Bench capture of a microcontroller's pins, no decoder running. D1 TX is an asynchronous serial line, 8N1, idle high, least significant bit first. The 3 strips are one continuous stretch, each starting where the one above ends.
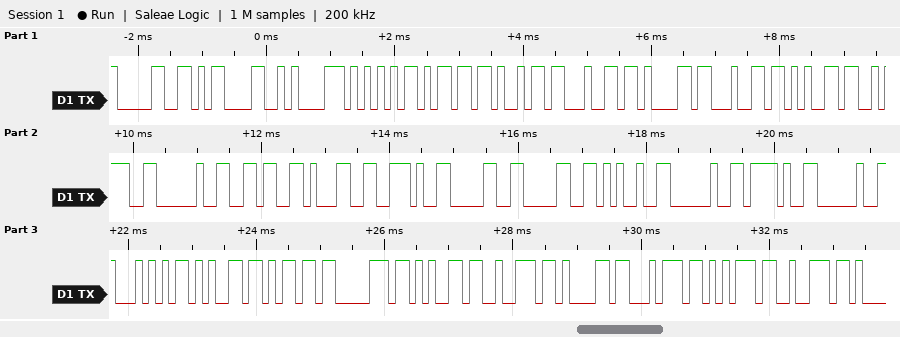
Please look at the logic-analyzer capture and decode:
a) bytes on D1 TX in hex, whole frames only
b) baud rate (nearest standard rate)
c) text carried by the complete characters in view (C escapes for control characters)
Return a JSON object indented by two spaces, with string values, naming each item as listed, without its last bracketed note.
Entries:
{
  "bytes on D1 TX in hex, whole frames only": "30 0D 0A 55 6D 69 64 61 64 65 3A 20 36 31 2E 30 30 25 20 2F 20 54 65 6D 70 65 72 61 74 75 72",
  "baud rate": "9600 baud",
  "text carried by the complete characters in view": "\"0\\r\\nUmidade: 61.00% / Temperatur\""
}
